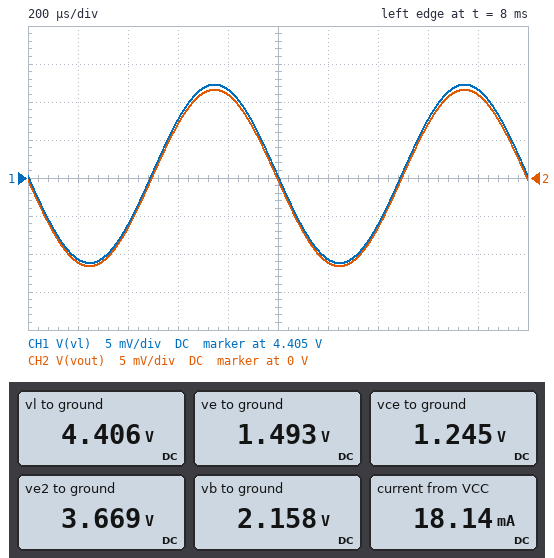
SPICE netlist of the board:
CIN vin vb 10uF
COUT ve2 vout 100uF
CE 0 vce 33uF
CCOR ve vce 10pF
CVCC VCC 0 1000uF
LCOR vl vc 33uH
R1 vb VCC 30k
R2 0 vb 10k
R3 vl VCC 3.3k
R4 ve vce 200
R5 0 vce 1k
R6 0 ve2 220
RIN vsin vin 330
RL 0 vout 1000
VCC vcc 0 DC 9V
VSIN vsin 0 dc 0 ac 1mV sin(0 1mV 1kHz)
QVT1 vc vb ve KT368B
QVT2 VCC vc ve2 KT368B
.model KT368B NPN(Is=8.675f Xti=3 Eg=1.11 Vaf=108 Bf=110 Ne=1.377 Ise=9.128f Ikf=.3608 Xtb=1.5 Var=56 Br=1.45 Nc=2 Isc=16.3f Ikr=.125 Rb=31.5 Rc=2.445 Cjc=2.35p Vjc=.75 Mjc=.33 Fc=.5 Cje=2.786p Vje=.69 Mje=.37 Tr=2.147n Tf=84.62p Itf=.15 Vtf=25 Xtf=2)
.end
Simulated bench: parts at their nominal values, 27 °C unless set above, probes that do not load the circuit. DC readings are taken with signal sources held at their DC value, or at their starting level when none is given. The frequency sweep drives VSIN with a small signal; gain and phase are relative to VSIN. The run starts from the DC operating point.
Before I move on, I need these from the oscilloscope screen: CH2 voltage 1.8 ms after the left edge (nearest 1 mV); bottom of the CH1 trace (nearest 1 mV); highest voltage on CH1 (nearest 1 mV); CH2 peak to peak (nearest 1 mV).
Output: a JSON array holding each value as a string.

["11 mV", "4.394 V", "4.417 V", "23 mV"]
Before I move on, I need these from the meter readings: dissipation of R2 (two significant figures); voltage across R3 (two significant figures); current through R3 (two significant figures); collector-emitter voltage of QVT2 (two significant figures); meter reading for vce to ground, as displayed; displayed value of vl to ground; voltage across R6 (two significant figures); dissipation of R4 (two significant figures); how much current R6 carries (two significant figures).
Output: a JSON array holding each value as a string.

["470 µW", "4.6 V", "1.4 mA", "5.3 V", "1.245 V", "4.406 V", "3.7 V", "310 µW", "17 mA"]
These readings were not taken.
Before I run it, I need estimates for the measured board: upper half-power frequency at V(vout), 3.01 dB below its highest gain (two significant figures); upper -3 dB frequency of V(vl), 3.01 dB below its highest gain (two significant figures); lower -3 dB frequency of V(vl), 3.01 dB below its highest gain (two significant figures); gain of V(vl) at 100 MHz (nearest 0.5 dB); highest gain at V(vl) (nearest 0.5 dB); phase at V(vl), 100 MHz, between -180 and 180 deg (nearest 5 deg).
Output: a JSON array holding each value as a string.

["17 MHz", "13 MHz", "26 Hz", "-12.5 dB", "21.5 dB", "10 deg"]
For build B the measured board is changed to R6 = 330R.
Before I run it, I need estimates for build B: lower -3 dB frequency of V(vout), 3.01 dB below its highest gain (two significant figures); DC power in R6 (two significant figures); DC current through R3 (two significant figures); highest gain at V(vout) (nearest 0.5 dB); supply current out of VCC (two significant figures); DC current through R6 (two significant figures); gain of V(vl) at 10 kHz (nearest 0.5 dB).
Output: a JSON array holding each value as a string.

["32 Hz", "45 mW", "1.3 mA", "22.5 dB", "13 mA", "12 mA", "22.0 dB"]
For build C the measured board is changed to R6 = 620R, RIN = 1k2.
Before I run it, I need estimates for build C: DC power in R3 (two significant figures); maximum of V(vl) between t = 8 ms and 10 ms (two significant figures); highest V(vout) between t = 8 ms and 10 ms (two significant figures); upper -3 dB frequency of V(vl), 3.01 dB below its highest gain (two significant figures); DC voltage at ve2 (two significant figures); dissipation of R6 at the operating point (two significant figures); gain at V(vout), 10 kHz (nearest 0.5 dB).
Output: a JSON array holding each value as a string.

["5.5 mW", "4.7 V", "11 mV", "7.0 MHz", "4.0 V", "26 mW", "21.0 dB"]
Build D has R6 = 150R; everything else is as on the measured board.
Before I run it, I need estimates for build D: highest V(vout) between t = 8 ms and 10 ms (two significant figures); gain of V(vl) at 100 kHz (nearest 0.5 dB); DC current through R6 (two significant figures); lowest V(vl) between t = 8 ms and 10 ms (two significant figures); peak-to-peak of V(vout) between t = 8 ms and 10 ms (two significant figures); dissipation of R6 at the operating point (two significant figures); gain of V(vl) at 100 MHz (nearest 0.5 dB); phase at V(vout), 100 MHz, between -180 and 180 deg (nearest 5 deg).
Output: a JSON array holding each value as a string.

["11 mV", "21.0 dB", "23 mA", "4.2 V", "22 mV", "79 mW", "-13.0 dB", "90 deg"]
